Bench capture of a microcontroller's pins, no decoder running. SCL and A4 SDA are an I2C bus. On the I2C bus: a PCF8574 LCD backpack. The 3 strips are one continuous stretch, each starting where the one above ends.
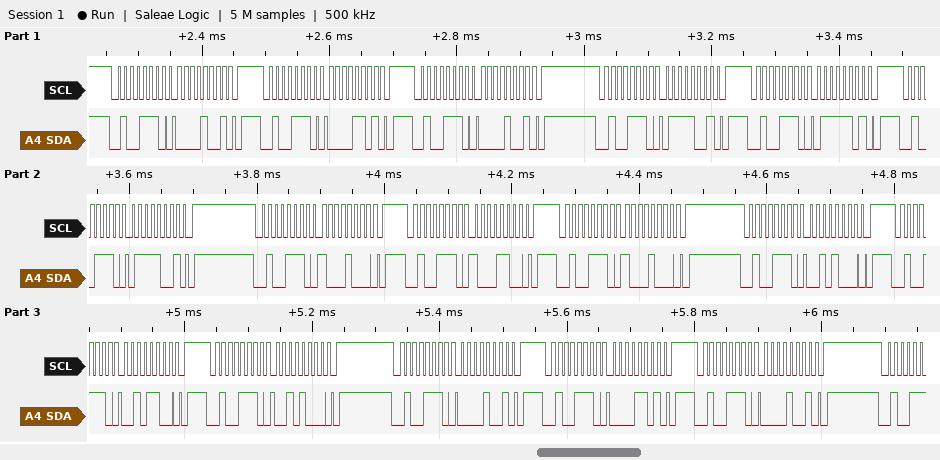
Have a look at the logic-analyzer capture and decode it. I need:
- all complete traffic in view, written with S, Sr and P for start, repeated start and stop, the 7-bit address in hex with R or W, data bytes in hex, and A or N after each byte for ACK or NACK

S 27W A 09 A P S 27W A 0D A P S 27W A 09 A P S 27W A 79 A P S 27W A 7D A P S 27W A 79 A P S 27W A 88 A P S 27W A 8C A P S 27W A 88 A P S 27W A 28 A P S 27W A 2C A P S 27W A 28 A P S 27W A 09 A P S 27W A 0D A P S 27W A 09 A P
